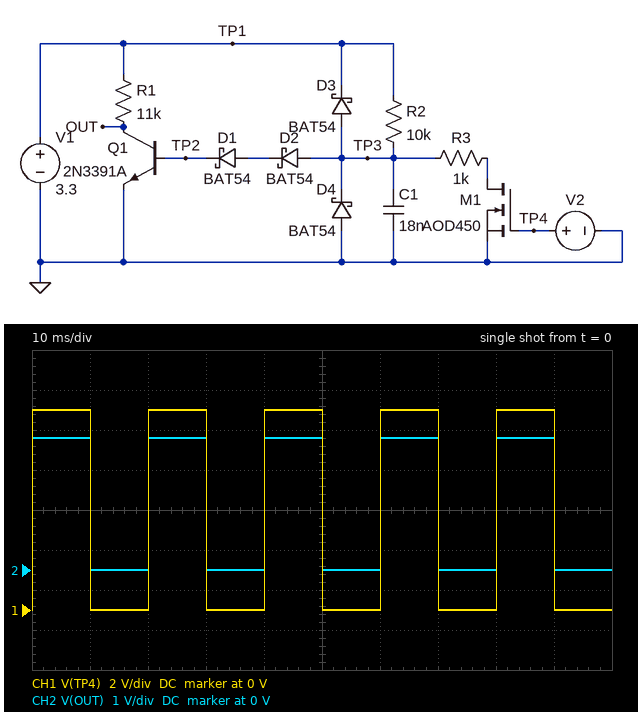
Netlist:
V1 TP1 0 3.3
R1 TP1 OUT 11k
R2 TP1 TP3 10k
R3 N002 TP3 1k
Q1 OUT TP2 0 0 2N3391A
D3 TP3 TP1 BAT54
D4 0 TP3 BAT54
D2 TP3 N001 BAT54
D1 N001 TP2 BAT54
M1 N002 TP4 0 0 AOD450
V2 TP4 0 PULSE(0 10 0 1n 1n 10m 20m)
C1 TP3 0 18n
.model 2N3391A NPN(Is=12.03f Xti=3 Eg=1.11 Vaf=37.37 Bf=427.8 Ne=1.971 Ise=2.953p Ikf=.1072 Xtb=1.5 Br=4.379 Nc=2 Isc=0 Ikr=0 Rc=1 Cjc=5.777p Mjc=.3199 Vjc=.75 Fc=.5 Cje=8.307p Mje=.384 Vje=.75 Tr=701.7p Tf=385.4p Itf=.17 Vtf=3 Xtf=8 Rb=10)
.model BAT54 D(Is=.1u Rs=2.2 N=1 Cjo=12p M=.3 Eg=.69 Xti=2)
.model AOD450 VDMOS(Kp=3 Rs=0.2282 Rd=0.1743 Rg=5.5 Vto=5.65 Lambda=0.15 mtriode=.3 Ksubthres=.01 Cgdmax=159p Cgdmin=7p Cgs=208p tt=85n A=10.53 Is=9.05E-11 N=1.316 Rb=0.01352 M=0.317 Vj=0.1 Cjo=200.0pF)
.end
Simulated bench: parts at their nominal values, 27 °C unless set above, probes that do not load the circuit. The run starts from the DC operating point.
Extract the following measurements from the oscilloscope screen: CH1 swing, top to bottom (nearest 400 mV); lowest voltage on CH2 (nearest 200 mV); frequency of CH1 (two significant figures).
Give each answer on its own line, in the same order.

10.0 V
0 V
50 Hz
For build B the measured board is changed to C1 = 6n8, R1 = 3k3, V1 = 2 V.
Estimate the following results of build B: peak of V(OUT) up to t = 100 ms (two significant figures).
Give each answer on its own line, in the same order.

2.0 V
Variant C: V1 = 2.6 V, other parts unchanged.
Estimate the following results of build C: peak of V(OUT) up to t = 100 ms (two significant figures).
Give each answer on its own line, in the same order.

2.6 V
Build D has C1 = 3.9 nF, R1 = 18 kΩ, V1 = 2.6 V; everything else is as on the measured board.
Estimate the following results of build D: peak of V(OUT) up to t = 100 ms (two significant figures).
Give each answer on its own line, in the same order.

2.6 V
